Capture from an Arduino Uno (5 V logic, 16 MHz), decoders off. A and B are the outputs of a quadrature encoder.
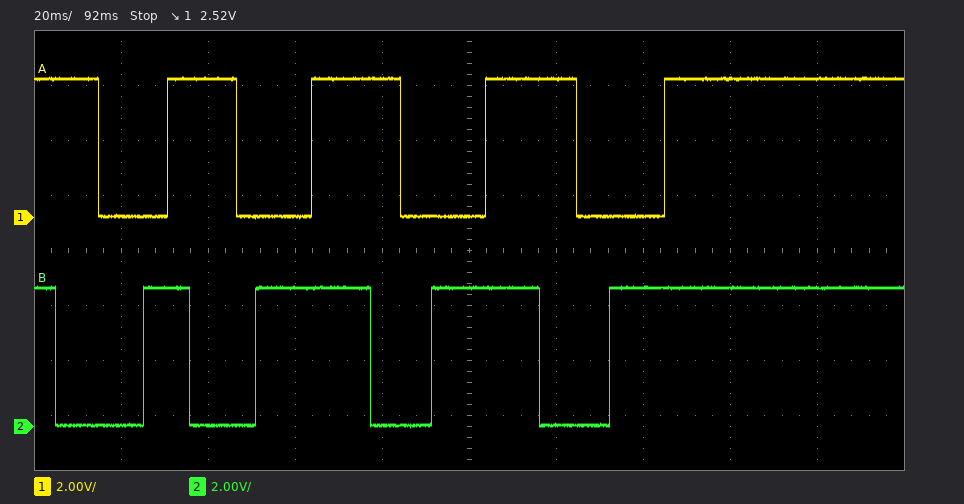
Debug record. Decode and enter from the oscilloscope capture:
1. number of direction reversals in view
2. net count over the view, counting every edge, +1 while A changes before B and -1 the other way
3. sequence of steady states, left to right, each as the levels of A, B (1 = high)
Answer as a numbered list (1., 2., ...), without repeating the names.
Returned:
1. 0
2. -16
3. 11 10 00 01 11 10 00 01 11 10 00 01 11 10 00 01 11
